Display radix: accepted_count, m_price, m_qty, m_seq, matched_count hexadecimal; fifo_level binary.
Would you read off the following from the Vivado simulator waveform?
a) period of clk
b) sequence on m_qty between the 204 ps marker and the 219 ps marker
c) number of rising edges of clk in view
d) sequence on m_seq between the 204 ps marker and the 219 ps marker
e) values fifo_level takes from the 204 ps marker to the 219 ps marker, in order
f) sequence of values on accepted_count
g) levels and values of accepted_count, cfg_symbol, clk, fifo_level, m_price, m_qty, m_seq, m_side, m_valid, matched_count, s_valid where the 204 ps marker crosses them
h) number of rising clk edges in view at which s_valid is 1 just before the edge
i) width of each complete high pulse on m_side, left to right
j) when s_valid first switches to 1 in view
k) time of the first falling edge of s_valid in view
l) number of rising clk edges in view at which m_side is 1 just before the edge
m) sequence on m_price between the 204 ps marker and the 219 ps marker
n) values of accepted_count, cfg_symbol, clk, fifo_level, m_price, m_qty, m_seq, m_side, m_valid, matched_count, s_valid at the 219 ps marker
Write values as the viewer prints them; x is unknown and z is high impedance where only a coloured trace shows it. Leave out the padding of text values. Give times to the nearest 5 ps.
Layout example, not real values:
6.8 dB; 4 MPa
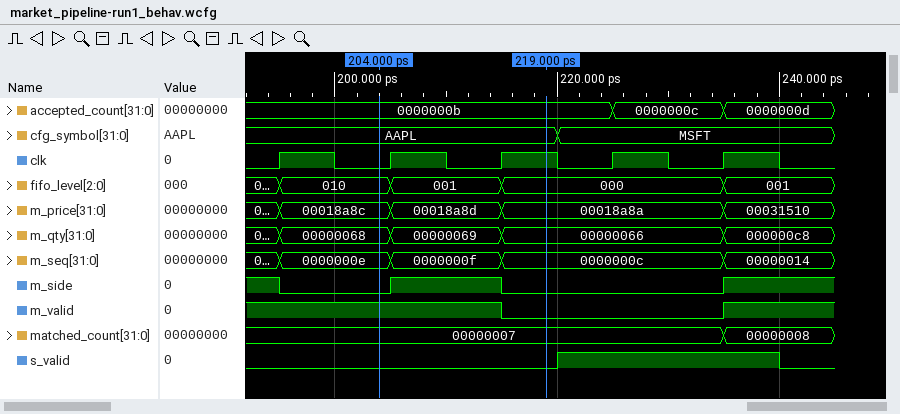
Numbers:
10 ps; 00000068, 00000069, 00000066; 5; 0000000e, 0000000f, 0000000c; 010, 001, 000; 0000000b, 0000000c, 0000000d; accepted_count=0000000b, cfg_symbol=AAPL, clk=0, fifo_level=010, m_price=00018a8c, m_qty=00000068, m_seq=0000000e, m_side=0, m_valid=1, matched_count=00000007, s_valid=0; 2; 10 ps; 220 ps; 240 ps; 2; 00018a8c, 00018a8d, 00018a8a; accepted_count=0000000b, cfg_symbol=AAPL, clk=1, fifo_level=000, m_price=00018a8a, m_qty=00000066, m_seq=0000000c, m_side=0, m_valid=0, matched_count=00000007, s_valid=0
